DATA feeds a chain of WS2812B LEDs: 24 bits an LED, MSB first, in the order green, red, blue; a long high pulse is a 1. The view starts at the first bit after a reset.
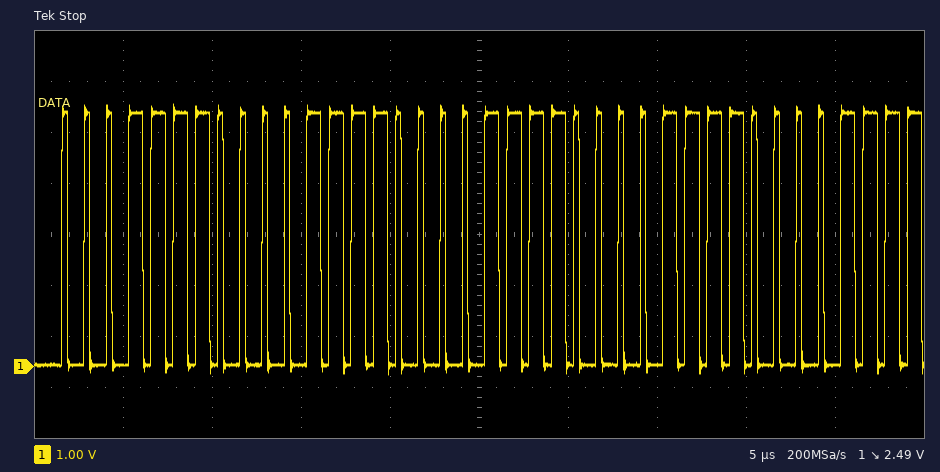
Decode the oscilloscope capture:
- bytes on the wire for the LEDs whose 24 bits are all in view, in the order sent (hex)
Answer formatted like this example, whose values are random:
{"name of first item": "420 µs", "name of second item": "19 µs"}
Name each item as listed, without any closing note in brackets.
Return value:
{"bytes on the wire for the LEDs whose 24 bits are all in view, in the order sent": "1E 1E 1E"}
